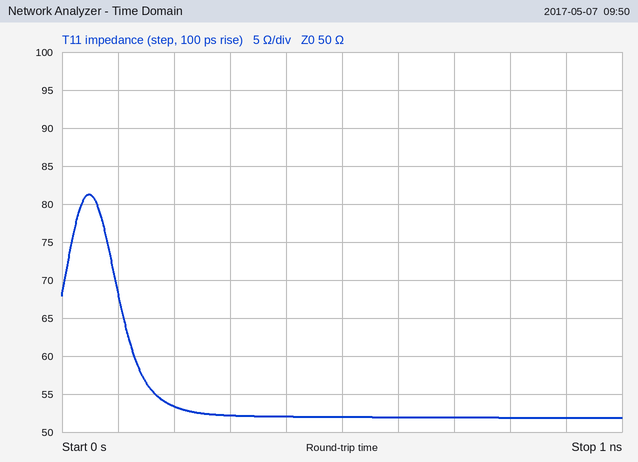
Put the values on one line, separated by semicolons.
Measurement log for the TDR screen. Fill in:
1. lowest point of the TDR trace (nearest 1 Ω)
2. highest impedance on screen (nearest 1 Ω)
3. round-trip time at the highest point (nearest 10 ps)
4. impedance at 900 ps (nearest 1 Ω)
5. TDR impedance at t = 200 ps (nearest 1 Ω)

52 Ω; 81 Ω; 50 ps; 52 Ω; 53 Ω
